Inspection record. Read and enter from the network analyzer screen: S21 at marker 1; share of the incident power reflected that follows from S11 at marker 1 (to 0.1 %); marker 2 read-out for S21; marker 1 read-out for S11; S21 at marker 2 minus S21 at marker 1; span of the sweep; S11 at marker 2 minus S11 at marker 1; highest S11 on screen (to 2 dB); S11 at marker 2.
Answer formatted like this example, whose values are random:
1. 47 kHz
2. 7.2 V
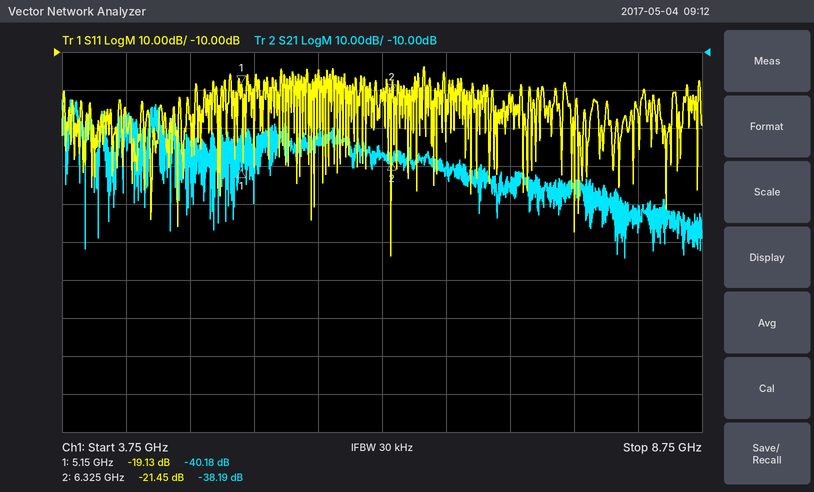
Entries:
1. -40.18 dB
2. 1.2 %
3. -38.19 dB
4. -19.13 dB
5. 1.99 dB
6. 5 GHz
7. -2.32 dB
8. -14 dB
9. -21.45 dB
